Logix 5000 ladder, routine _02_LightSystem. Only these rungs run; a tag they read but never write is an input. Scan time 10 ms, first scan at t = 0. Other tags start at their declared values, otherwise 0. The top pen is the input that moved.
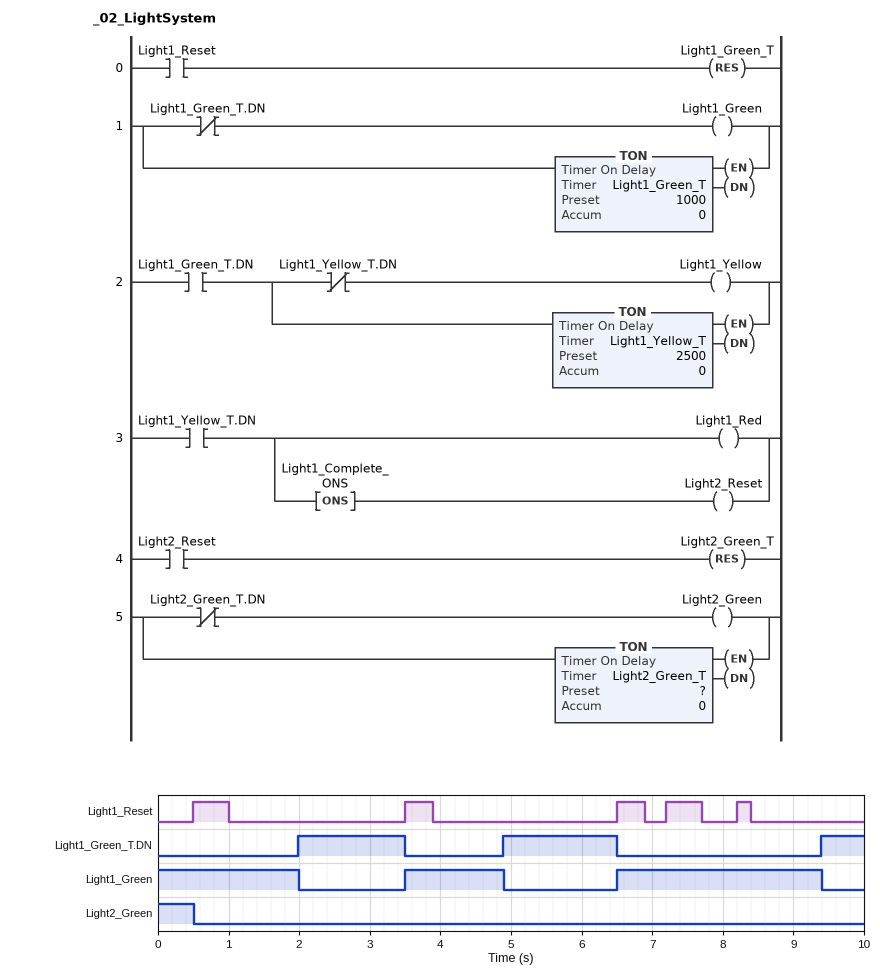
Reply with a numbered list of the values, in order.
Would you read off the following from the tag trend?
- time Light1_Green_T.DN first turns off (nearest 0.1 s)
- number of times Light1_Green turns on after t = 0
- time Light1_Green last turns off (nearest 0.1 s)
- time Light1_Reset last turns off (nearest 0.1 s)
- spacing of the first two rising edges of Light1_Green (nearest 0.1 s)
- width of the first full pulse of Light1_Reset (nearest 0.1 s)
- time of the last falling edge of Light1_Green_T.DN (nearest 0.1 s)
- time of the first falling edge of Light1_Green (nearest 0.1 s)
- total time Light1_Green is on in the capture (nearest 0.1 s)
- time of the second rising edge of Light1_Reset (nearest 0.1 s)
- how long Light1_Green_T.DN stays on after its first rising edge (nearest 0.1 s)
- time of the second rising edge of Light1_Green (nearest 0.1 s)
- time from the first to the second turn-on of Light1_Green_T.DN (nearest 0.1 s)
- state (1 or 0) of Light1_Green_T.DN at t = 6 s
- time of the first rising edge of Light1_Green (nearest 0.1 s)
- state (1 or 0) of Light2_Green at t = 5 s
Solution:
1. 3.5 s
2. 2
3. 9.4 s
4. 8.4 s
5. 3.0 s
6. 0.5 s
7. 6.5 s
8. 2.0 s
9. 6.3 s
10. 3.5 s
11. 1.5 s
12. 6.5 s
13. 2.9 s
14. 1
15. 3.5 s
16. 0
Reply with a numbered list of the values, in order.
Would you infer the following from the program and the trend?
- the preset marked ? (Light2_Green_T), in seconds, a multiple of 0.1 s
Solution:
1. 0.5 s
